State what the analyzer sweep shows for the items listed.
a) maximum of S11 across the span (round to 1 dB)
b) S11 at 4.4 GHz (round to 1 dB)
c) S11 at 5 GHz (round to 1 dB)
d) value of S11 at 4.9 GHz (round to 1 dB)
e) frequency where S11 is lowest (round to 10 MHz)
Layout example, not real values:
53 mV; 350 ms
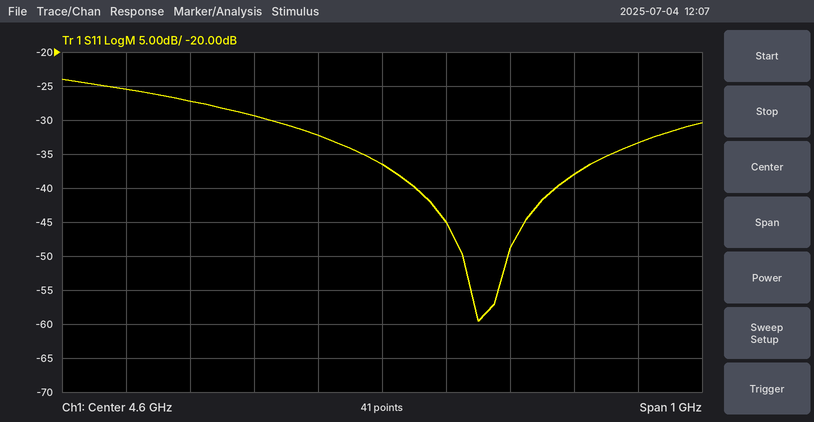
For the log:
-24 dB; -29 dB; -33 dB; -38 dB; 4.75 GHz
